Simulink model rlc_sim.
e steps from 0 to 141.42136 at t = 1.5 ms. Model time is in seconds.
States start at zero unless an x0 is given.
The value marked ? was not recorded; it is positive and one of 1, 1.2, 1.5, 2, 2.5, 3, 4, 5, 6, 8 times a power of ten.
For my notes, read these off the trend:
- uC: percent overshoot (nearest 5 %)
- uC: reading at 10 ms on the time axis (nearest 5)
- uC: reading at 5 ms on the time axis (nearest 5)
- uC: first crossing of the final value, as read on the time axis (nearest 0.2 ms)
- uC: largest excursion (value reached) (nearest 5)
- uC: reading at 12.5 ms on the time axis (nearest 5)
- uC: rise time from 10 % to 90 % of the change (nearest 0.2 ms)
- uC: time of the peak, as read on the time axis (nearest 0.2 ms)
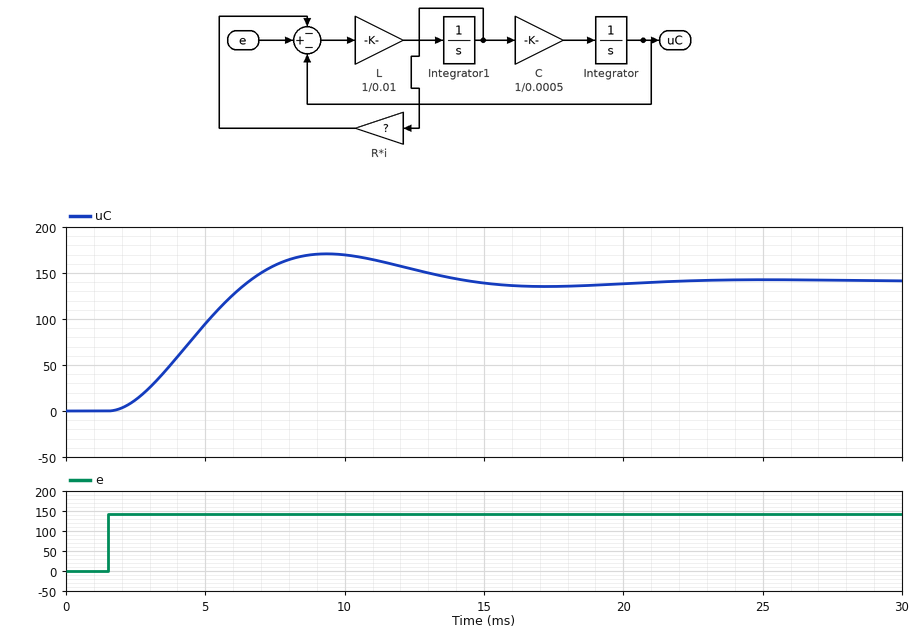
20 %
170
95
6.6 ms
170
155
3.4 ms
9.4 ms
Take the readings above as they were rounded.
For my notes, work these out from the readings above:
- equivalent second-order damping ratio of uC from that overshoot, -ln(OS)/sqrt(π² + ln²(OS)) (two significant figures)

0.46
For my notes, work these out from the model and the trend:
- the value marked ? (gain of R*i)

4
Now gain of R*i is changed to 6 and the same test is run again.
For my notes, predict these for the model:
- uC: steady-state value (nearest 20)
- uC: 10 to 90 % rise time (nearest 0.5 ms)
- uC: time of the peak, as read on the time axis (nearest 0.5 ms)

140
4.5 ms
11.0 ms
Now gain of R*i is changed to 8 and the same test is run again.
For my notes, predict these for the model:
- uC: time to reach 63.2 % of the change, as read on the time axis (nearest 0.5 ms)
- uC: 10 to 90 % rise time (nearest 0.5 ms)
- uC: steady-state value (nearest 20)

6.0 ms
6.5 ms
140
